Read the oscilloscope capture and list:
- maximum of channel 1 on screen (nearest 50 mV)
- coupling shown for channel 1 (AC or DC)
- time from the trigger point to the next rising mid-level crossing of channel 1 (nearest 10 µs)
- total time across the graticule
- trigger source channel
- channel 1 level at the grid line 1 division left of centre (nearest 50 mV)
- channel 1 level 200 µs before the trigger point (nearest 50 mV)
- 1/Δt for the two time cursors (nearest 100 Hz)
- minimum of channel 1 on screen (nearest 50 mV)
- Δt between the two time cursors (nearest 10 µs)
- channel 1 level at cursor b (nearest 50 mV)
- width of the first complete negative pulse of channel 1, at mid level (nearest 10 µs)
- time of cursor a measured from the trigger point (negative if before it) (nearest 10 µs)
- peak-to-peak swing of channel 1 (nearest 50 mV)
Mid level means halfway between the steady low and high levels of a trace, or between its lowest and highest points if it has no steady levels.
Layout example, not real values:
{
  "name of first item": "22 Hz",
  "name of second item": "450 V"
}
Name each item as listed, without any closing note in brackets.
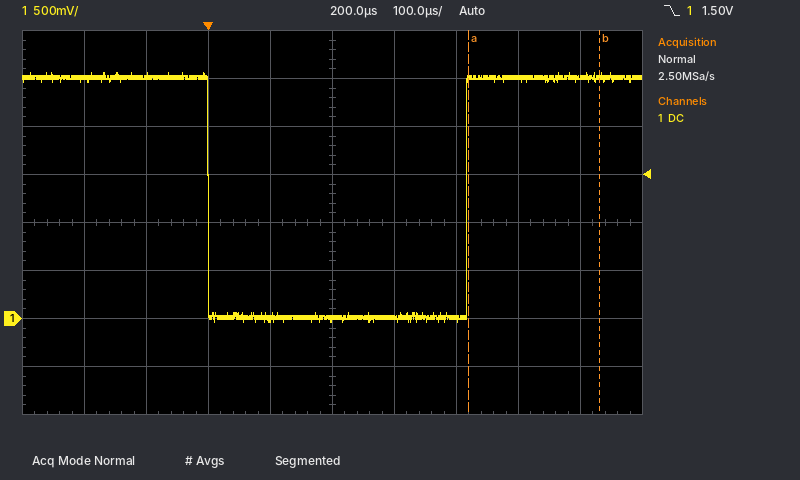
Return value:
{
  "maximum of channel 1 on screen": "2.55 V",
  "coupling shown for channel 1": "DC",
  "time from the trigger point to the next rising mid-level crossing of channel 1": "420 µs",
  "total time across the graticule": "1 ms",
  "trigger source channel": "channel 1",
  "channel 1 level at the grid line 1 division left of centre": "0 mV",
  "channel 1 level 200 µs before the trigger point": "2.50 V",
  "1/Δt for the two time cursors": "4.8 kHz",
  "minimum of channel 1 on screen": "-50 mV",
  "Δt between the two time cursors": "210 µs",
  "channel 1 level at cursor b": "2.55 V",
  "width of the first complete negative pulse of channel 1, at mid level": "420 µs",
  "time of cursor a measured from the trigger point (negative if before it)": "+420 µs",
  "peak-to-peak swing of channel 1": "2.60 V"
}
